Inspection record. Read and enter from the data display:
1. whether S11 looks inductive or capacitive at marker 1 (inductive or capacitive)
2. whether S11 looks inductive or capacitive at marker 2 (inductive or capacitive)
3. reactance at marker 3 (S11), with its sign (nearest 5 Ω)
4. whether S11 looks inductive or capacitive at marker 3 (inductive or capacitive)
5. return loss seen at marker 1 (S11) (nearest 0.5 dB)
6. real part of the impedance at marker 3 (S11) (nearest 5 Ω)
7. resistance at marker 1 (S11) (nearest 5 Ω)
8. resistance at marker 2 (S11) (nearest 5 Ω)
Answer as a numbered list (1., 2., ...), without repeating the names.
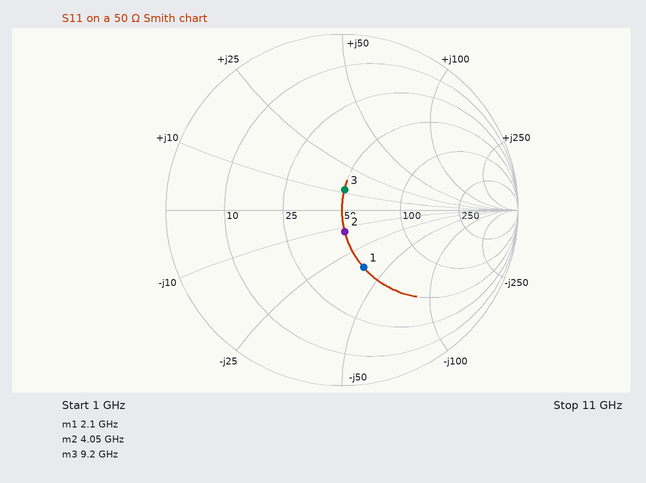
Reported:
1. capacitive
2. capacitive
3. +10 Ω
4. inductive
5. 9.0 dB
6. 50 Ω
7. 50 Ω
8. 50 Ω
